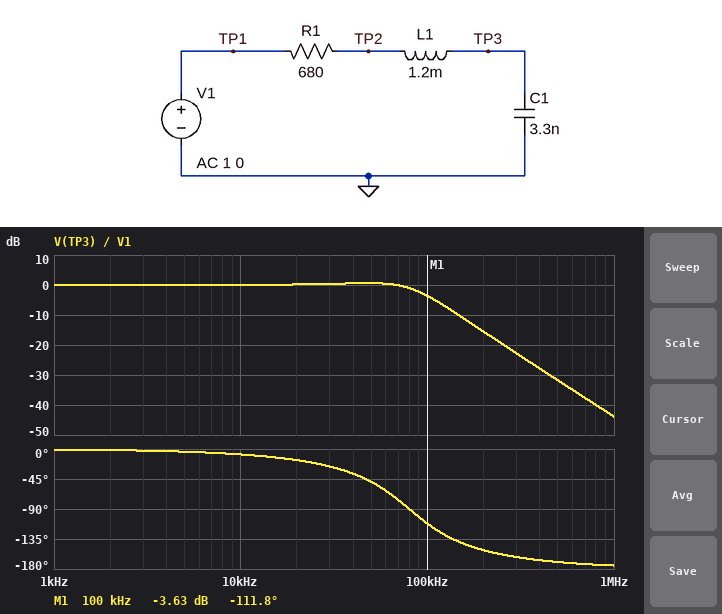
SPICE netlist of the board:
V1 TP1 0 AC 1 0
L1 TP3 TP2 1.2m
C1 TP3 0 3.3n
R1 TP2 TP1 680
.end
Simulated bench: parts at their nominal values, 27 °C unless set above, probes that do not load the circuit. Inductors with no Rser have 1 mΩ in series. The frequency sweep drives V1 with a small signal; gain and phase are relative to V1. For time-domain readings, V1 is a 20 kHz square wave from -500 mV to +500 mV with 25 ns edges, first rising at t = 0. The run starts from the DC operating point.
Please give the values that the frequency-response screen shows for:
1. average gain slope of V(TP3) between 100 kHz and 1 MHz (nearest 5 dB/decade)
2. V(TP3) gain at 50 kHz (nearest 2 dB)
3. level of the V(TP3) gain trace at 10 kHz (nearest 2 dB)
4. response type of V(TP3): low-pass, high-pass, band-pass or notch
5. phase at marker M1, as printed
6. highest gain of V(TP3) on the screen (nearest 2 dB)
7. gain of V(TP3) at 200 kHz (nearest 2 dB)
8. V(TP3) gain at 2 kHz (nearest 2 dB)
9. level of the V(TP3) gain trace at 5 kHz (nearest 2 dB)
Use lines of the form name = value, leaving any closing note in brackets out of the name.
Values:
average gain slope of V(TP3) between 100 kHz and 1 MHz = -40 dB/decade
V(TP3) gain at 50 kHz = 0 dB
level of the V(TP3) gain trace at 10 kHz = 0 dB
response type of V(TP3): low-pass, high-pass, band-pass or notch = low-pass
phase at marker M1, as printed = -111.8 deg
highest gain of V(TP3) on the screen = 0 dB
gain of V(TP3) at 200 kHz = -16 dB
V(TP3) gain at 2 kHz = 0 dB
level of the V(TP3) gain trace at 5 kHz = 0 dB
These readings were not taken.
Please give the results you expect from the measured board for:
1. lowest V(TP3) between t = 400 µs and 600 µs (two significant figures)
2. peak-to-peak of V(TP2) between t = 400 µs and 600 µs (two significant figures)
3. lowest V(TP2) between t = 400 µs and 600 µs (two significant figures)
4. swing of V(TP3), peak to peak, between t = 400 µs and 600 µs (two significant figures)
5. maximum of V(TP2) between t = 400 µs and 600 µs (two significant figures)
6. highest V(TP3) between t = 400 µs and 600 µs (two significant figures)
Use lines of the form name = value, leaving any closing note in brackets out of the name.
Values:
lowest V(TP3) between t = 400 µs and 600 µs = -620 mV
peak-to-peak of V(TP2) between t = 400 µs and 600 µs = 1.1 V
lowest V(TP2) between t = 400 µs and 600 µs = -570 mV
swing of V(TP3), peak to peak, between t = 400 µs and 600 µs = 1.2 V
maximum of V(TP2) between t = 400 µs and 600 µs = 570 mV
highest V(TP3) between t = 400 µs and 600 µs = 620 mV
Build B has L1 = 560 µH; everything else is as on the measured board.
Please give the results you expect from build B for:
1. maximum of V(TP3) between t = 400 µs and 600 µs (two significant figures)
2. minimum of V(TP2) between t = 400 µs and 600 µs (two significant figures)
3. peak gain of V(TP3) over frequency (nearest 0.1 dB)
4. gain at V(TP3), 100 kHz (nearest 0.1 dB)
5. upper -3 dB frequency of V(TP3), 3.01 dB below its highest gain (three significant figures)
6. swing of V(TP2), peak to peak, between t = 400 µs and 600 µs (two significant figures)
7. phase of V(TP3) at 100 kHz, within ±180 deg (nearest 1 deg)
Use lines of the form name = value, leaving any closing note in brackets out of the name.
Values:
maximum of V(TP3) between t = 400 µs and 600 µs = 510 mV
minimum of V(TP2) between t = 400 µs and 600 µs = -510 mV
peak gain of V(TP3) over frequency = 0 dB
gain at V(TP3), 100 kHz = -3.1 dB
upper -3 dB frequency of V(TP3), 3.01 dB below its highest gain = 98.0 kHz
swing of V(TP2), peak to peak, between t = 400 µs and 600 µs = 1.0 V
phase of V(TP3) at 100 kHz, within ±180 deg = -79 deg
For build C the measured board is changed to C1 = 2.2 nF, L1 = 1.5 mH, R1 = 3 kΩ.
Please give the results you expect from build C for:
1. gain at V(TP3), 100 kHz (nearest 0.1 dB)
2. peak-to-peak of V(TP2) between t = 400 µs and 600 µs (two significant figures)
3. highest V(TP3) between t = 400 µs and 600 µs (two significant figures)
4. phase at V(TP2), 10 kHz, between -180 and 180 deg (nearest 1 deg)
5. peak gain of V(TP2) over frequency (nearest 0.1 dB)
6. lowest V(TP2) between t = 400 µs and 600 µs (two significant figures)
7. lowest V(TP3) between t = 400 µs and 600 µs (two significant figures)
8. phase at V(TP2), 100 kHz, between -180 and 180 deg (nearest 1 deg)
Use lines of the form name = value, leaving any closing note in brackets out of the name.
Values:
gain at V(TP3), 100 kHz = -12.4 dB
peak-to-peak of V(TP2) between t = 400 µs and 600 µs = 990 mV
highest V(TP3) between t = 400 µs and 600 µs = 480 mV
phase at V(TP2), 10 kHz, between -180 and 180 deg = -23 deg
peak gain of V(TP2) over frequency = 0 dB
lowest V(TP2) between t = 400 µs and 600 µs = -490 mV
lowest V(TP3) between t = 400 µs and 600 µs = -480 mV
phase at V(TP2), 100 kHz, between -180 and 180 deg = 86 deg
